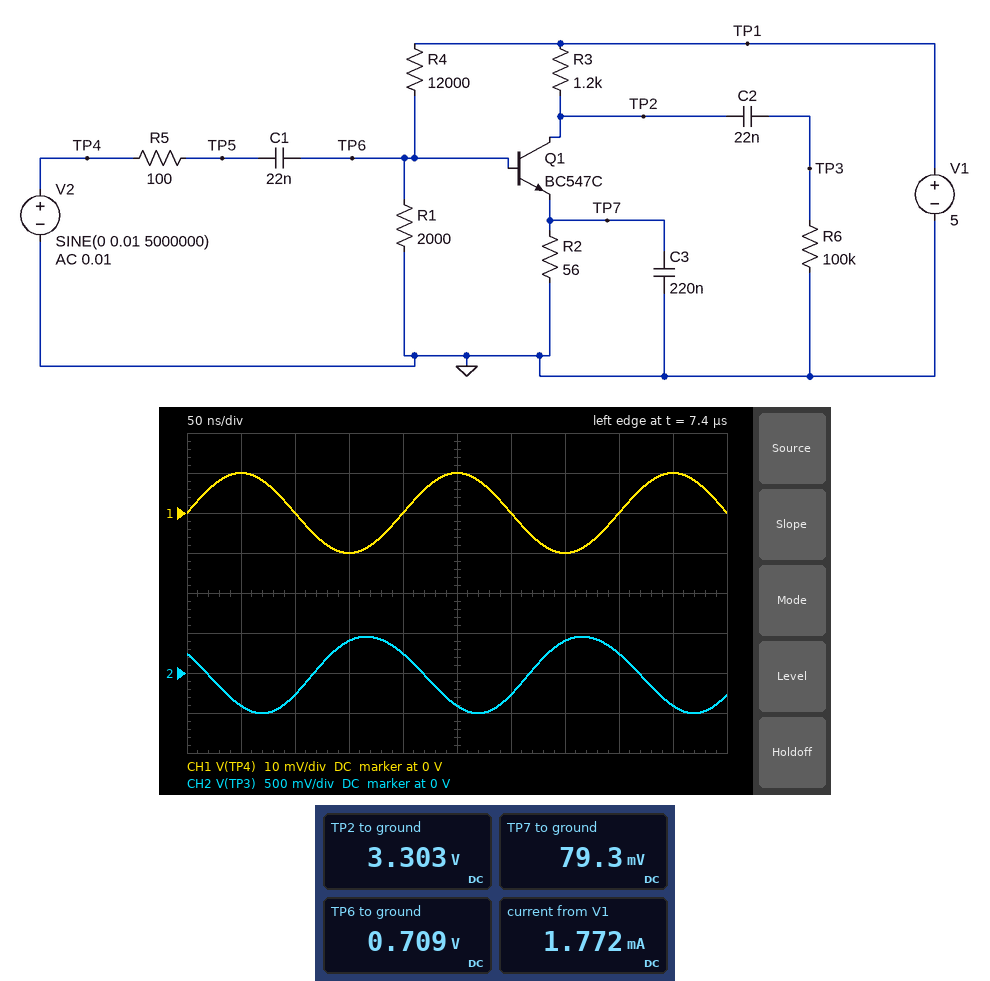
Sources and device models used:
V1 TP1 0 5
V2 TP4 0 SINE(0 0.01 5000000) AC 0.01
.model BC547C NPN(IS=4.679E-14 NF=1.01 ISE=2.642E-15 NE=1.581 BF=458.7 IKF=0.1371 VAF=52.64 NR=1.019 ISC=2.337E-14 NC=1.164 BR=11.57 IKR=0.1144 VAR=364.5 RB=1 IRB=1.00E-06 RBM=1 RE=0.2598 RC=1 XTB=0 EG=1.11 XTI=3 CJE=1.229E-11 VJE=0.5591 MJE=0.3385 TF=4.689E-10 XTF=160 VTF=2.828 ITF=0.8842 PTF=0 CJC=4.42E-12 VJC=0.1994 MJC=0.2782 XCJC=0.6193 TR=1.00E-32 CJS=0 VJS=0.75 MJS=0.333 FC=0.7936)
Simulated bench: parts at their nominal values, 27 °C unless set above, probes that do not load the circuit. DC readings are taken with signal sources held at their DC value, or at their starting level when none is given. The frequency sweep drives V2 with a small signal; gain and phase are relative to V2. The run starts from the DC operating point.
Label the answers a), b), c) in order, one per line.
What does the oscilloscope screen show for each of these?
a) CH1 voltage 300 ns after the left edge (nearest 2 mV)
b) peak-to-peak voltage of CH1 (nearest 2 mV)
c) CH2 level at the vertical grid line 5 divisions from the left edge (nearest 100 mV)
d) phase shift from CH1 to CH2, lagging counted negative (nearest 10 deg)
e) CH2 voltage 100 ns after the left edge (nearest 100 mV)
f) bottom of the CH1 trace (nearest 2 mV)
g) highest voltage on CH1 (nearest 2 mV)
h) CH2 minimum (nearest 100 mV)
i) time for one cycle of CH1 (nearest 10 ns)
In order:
a) 0 V
b) 20 mV
c) -400 mV
d) 150 deg
e) -300 mV
f) -10 mV
g) 10 mV
h) -500 mV
i) 200 ns
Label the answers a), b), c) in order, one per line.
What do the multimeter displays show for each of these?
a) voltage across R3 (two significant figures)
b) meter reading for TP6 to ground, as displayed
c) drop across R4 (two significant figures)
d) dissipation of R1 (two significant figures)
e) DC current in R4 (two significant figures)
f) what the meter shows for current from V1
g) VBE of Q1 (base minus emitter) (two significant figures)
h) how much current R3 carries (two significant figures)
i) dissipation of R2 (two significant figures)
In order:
a) 1.7 V
b) 0.709 V
c) 4.3 V
d) 250 µW
e) 360 µA
f) 1.772 mA
g) 630 mV
h) 1.4 mA
i) 110 µW
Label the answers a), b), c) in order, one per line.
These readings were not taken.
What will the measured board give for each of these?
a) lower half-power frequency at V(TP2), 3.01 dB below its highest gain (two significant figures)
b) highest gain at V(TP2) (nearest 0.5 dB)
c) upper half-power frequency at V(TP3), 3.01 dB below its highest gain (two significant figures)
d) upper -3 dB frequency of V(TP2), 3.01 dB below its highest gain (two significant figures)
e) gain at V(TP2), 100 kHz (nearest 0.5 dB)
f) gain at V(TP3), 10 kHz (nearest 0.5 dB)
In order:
a) 47 kHz
b) 35.0 dB
c) 8.3 MHz
d) 8.3 MHz
e) 34.0 dB
f) 24.5 dB
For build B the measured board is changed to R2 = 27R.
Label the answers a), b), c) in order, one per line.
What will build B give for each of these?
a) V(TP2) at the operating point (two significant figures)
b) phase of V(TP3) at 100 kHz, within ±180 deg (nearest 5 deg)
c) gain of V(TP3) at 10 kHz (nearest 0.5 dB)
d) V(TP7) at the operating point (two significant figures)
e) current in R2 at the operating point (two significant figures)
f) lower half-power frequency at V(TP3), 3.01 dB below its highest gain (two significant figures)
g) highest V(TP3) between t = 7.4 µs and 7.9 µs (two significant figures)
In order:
a) 2.2 V
b) -155 deg
c) 28.5 dB
d) 62 mV
e) 2.3 mA
f) 74 kHz
g) 620 mV
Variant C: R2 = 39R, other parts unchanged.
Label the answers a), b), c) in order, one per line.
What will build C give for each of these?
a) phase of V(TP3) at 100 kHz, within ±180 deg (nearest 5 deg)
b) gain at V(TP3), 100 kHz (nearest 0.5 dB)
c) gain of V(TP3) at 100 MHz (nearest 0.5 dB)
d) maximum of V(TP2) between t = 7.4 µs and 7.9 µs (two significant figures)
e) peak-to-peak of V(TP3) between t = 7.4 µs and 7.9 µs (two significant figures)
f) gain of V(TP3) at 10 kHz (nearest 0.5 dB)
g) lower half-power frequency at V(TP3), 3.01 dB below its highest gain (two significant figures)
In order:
a) -155 deg
b) 35.5 dB
c) 13.0 dB
d) 3.4 V
e) 1.1 V
f) 26.5 dB
g) 59 kHz
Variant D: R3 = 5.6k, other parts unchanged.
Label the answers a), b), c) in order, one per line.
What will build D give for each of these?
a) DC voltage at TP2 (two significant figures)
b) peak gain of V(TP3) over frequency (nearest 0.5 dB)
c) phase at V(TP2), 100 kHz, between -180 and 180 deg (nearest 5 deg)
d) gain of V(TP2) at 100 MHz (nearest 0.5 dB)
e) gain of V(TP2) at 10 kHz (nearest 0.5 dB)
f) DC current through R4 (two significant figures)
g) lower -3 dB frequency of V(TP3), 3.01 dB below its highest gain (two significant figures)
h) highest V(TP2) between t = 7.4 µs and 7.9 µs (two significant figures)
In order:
a) 94 mV
b) 9.5 dB
c) -165 deg
d) -10.0 dB
e) 0.5 dB
f) 360 µA
g) 27 kHz
h) 150 mV
